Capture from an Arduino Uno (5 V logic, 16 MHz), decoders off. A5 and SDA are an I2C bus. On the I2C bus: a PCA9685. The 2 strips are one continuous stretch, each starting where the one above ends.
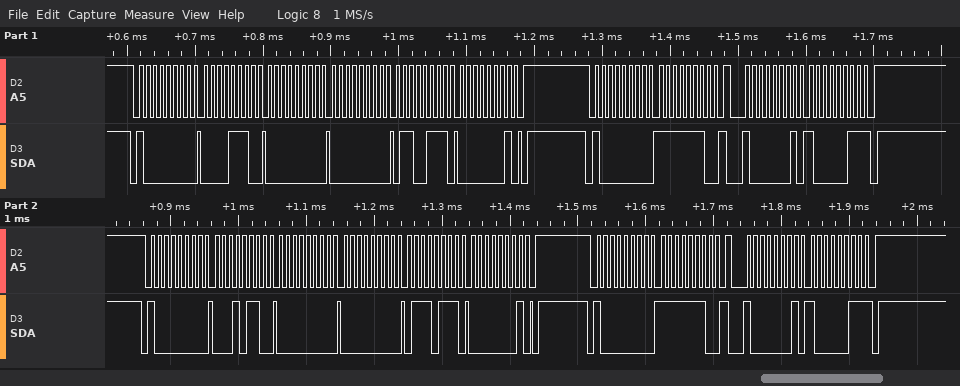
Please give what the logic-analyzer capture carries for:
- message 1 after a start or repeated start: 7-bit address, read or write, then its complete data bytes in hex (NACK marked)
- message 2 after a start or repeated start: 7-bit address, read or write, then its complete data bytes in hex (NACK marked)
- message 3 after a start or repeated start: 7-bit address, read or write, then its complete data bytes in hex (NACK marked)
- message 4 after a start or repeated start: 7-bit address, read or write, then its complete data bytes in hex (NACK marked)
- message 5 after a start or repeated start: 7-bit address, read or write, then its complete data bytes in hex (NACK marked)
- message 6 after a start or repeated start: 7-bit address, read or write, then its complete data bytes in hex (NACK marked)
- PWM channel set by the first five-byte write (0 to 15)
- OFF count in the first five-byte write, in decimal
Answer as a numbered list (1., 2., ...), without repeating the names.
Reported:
1. 0x40 write: 0E 00 00 67 01
2. 0x40 write: FE
3. 0x40 read: 83 NACK
4. 0x40 write: 16 00 00 77 01
5. 0x40 write: FE
6. 0x40 read: 83 NACK
7. 2
8. 359
